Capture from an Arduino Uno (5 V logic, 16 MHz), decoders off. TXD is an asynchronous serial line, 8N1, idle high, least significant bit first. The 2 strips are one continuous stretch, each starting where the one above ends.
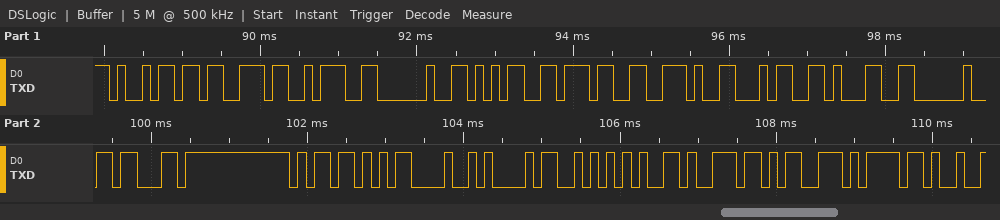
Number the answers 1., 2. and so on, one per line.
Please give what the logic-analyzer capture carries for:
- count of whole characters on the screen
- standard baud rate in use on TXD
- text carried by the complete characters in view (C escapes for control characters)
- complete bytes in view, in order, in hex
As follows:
1. 19
2. 9600 baud
3. "is: 57.41 cm\r\nSenso"
4. 0x69 0x73 0x3A 0x20 0x35 0x37 0x2E 0x34 0x31 0x20 0x63 0x6D 0x0D 0x0A 0x53 0x65 0x6E 0x73 0x6F
